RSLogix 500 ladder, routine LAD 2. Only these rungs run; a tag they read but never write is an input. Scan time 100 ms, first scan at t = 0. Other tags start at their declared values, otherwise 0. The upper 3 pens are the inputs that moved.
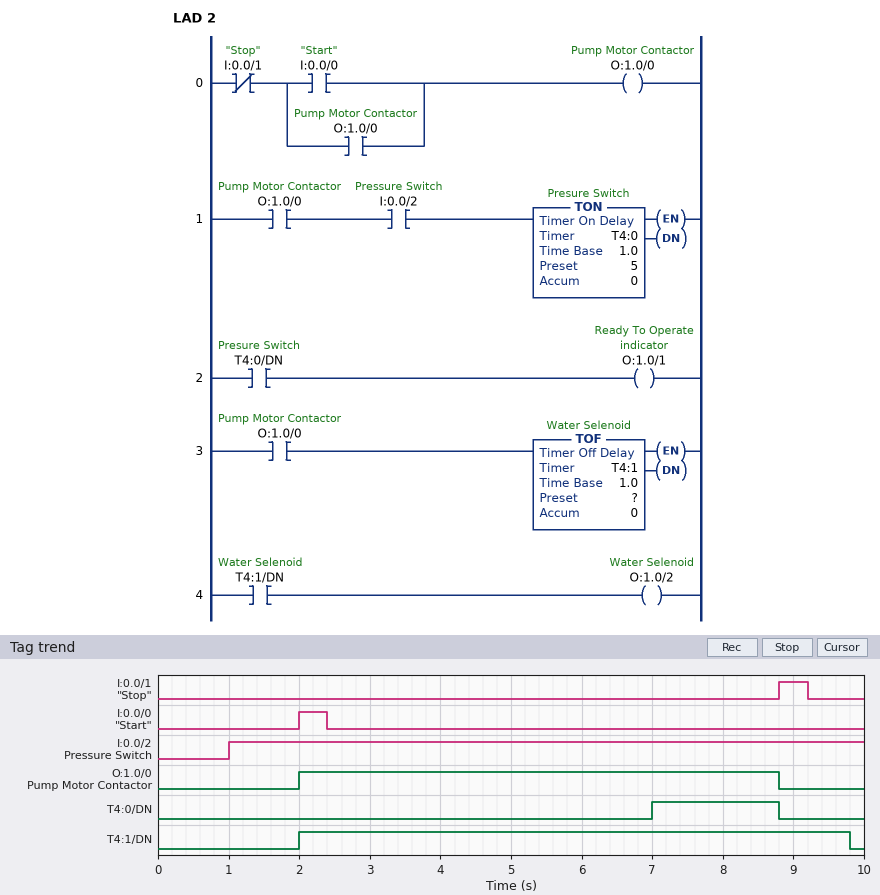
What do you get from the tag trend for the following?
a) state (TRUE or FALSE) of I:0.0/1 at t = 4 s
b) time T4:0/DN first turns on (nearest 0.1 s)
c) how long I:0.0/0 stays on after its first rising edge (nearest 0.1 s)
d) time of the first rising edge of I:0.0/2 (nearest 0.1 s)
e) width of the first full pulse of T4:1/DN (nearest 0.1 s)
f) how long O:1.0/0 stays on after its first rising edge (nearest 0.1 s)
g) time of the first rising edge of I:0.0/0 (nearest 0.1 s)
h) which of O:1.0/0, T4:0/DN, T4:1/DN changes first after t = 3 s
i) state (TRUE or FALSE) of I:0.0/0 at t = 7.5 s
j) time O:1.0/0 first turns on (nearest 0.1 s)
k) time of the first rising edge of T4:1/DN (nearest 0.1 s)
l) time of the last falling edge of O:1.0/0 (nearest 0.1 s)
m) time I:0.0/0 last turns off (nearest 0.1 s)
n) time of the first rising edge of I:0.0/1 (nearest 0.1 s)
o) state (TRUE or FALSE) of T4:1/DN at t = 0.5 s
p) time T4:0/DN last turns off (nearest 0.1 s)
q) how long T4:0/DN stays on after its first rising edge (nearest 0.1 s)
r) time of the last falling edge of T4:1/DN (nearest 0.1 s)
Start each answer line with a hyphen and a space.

- FALSE
- 7.0 s
- 0.4 s
- 1.0 s
- 7.8 s
- 6.8 s
- 2.0 s
- T4:0/DN
- FALSE
- 2.0 s
- 2.0 s
- 8.8 s
- 2.4 s
- 8.8 s
- FALSE
- 8.8 s
- 1.8 s
- 9.8 s
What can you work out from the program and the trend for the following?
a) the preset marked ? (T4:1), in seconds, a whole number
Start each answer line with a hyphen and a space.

- 1 s
